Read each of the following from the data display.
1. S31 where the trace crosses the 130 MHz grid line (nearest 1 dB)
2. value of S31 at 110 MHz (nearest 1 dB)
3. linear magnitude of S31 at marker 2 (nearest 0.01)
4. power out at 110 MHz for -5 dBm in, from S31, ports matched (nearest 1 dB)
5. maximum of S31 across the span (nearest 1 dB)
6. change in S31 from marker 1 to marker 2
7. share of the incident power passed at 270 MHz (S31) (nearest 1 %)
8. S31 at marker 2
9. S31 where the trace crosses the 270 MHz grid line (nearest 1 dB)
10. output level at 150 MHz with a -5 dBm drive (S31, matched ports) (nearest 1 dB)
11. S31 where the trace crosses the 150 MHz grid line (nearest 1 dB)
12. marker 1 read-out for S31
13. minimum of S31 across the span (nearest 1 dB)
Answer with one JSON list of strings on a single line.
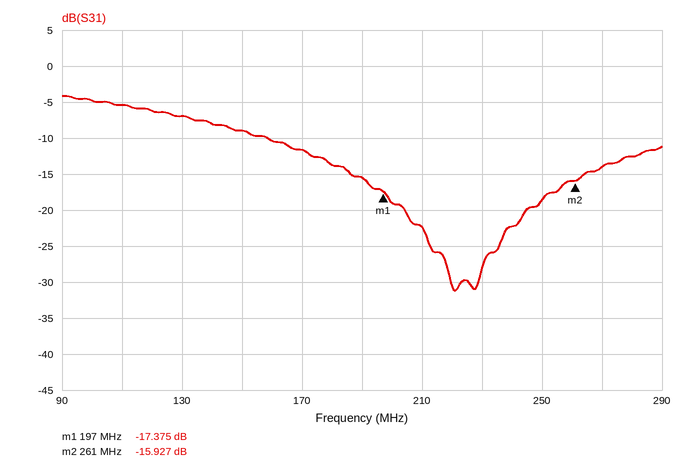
["-7 dB", "-5 dB", "0.16", "-10 dBm", "-4 dB", "1.448 dB", "4 %", "-15.927 dB", "-14 dB", "-14 dBm", "-9 dB", "-17.375 dB", "-31 dB"]
